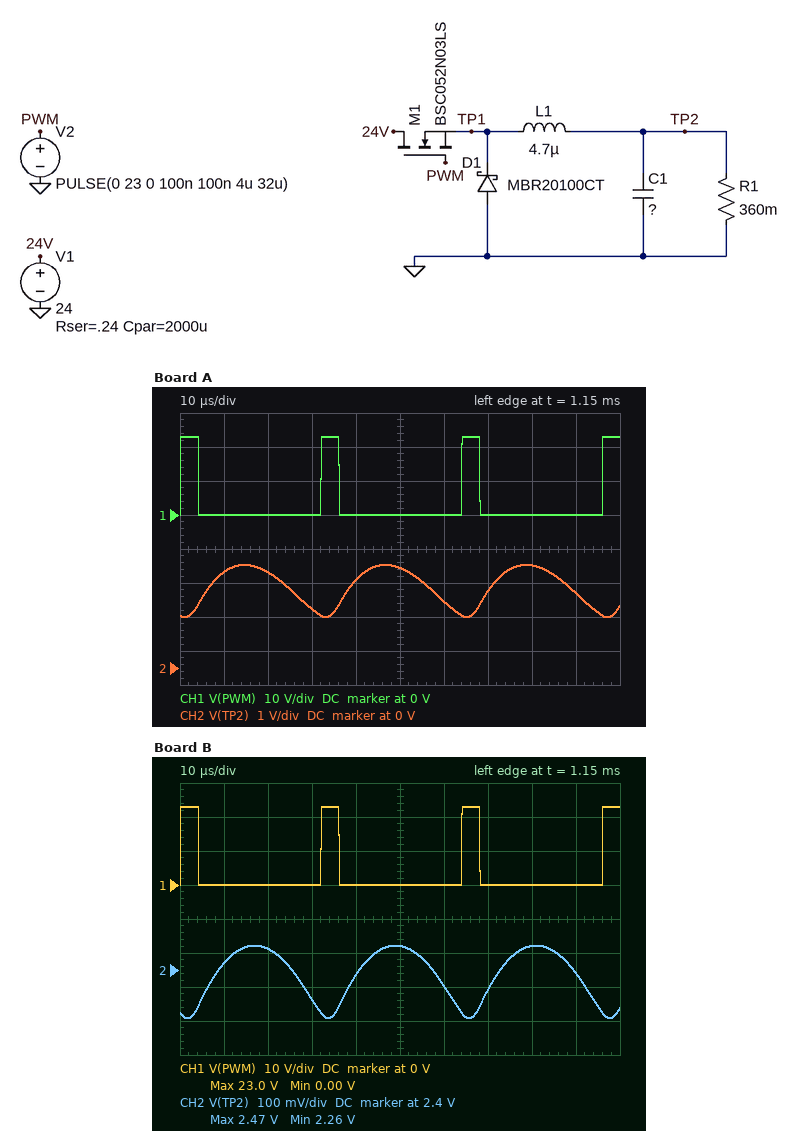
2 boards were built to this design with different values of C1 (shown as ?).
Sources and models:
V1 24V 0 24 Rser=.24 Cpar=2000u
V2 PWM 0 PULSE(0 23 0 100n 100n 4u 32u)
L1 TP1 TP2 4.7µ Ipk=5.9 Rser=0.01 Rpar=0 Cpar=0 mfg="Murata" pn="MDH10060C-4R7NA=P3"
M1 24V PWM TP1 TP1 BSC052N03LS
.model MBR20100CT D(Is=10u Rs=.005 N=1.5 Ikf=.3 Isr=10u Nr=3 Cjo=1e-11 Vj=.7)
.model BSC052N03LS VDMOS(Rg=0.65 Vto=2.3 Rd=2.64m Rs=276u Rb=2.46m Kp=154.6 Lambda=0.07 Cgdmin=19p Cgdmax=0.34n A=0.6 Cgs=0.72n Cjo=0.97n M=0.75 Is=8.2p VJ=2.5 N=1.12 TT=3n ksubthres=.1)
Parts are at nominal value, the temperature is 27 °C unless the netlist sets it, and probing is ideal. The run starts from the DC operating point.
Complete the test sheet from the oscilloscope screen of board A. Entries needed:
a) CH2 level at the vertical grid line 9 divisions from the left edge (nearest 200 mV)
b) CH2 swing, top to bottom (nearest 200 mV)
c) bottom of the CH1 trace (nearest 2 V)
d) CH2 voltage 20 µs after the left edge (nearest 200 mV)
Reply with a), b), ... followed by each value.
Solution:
a) 2.2 V
b) 1.6 V
c) 0 V
d) 2.8 V
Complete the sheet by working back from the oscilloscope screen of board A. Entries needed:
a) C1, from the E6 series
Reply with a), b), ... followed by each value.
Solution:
a) 47 µF
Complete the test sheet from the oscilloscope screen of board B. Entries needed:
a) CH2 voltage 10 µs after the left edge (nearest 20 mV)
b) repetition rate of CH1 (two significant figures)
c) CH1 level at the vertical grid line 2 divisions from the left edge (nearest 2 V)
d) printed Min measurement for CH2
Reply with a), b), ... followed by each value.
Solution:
a) 2.42 V
b) 31 kHz
c) 0 V
d) 2.26 V
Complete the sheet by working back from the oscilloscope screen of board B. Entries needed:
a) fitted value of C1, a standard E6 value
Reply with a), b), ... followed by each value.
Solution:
a) 330 µF
